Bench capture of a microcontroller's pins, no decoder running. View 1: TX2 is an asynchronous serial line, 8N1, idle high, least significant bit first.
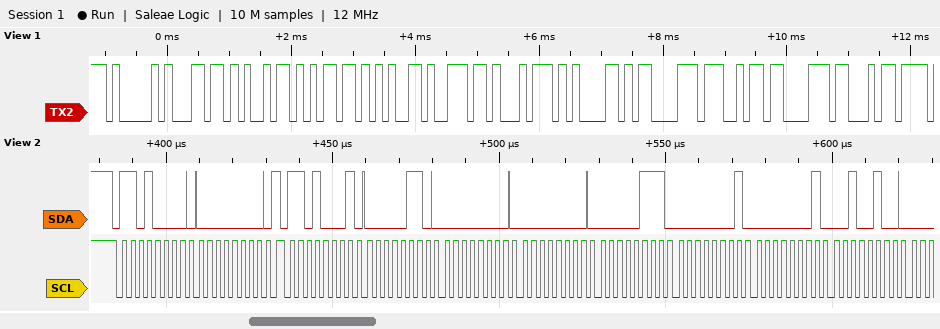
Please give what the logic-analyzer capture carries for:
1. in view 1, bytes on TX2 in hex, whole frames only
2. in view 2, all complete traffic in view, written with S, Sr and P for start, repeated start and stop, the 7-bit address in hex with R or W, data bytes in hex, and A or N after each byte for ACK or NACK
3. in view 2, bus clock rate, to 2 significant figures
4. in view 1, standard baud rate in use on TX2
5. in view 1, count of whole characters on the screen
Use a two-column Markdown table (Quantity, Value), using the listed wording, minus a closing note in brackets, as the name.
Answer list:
| Quantity | Value |
|---|---|
| in view 1, bytes on TX2 in hex, whole frames only | 41 6C 69 6D 65 6E 74 61 C3 A7 C3 A3 |
| in view 2, all complete traffic in view, written with S, Sr and P for start, repeated start and stop, the 7-bit address in hex with R or W, data bytes in hex, and A or N after each byte for ACK or NACK | S 68W A 00 A Sr 68R A 06 A 00 A 00 A 07 A 01 A 01 A 24 A |
| in view 2, bus clock rate, to 2 significant figures | 400 kHz |
| in view 1, standard baud rate in use on TX2 | 9600 baud |
| in view 1, count of whole characters on the screen | 12 |
